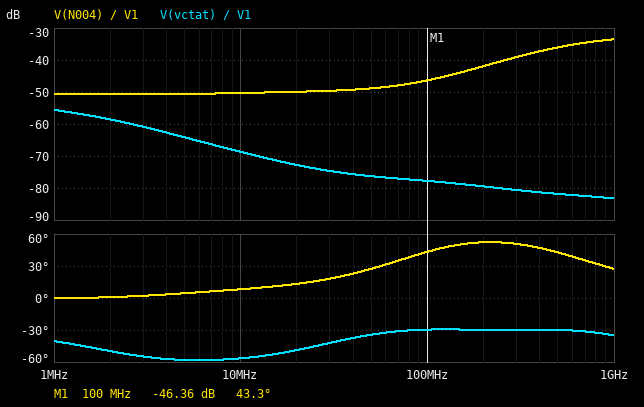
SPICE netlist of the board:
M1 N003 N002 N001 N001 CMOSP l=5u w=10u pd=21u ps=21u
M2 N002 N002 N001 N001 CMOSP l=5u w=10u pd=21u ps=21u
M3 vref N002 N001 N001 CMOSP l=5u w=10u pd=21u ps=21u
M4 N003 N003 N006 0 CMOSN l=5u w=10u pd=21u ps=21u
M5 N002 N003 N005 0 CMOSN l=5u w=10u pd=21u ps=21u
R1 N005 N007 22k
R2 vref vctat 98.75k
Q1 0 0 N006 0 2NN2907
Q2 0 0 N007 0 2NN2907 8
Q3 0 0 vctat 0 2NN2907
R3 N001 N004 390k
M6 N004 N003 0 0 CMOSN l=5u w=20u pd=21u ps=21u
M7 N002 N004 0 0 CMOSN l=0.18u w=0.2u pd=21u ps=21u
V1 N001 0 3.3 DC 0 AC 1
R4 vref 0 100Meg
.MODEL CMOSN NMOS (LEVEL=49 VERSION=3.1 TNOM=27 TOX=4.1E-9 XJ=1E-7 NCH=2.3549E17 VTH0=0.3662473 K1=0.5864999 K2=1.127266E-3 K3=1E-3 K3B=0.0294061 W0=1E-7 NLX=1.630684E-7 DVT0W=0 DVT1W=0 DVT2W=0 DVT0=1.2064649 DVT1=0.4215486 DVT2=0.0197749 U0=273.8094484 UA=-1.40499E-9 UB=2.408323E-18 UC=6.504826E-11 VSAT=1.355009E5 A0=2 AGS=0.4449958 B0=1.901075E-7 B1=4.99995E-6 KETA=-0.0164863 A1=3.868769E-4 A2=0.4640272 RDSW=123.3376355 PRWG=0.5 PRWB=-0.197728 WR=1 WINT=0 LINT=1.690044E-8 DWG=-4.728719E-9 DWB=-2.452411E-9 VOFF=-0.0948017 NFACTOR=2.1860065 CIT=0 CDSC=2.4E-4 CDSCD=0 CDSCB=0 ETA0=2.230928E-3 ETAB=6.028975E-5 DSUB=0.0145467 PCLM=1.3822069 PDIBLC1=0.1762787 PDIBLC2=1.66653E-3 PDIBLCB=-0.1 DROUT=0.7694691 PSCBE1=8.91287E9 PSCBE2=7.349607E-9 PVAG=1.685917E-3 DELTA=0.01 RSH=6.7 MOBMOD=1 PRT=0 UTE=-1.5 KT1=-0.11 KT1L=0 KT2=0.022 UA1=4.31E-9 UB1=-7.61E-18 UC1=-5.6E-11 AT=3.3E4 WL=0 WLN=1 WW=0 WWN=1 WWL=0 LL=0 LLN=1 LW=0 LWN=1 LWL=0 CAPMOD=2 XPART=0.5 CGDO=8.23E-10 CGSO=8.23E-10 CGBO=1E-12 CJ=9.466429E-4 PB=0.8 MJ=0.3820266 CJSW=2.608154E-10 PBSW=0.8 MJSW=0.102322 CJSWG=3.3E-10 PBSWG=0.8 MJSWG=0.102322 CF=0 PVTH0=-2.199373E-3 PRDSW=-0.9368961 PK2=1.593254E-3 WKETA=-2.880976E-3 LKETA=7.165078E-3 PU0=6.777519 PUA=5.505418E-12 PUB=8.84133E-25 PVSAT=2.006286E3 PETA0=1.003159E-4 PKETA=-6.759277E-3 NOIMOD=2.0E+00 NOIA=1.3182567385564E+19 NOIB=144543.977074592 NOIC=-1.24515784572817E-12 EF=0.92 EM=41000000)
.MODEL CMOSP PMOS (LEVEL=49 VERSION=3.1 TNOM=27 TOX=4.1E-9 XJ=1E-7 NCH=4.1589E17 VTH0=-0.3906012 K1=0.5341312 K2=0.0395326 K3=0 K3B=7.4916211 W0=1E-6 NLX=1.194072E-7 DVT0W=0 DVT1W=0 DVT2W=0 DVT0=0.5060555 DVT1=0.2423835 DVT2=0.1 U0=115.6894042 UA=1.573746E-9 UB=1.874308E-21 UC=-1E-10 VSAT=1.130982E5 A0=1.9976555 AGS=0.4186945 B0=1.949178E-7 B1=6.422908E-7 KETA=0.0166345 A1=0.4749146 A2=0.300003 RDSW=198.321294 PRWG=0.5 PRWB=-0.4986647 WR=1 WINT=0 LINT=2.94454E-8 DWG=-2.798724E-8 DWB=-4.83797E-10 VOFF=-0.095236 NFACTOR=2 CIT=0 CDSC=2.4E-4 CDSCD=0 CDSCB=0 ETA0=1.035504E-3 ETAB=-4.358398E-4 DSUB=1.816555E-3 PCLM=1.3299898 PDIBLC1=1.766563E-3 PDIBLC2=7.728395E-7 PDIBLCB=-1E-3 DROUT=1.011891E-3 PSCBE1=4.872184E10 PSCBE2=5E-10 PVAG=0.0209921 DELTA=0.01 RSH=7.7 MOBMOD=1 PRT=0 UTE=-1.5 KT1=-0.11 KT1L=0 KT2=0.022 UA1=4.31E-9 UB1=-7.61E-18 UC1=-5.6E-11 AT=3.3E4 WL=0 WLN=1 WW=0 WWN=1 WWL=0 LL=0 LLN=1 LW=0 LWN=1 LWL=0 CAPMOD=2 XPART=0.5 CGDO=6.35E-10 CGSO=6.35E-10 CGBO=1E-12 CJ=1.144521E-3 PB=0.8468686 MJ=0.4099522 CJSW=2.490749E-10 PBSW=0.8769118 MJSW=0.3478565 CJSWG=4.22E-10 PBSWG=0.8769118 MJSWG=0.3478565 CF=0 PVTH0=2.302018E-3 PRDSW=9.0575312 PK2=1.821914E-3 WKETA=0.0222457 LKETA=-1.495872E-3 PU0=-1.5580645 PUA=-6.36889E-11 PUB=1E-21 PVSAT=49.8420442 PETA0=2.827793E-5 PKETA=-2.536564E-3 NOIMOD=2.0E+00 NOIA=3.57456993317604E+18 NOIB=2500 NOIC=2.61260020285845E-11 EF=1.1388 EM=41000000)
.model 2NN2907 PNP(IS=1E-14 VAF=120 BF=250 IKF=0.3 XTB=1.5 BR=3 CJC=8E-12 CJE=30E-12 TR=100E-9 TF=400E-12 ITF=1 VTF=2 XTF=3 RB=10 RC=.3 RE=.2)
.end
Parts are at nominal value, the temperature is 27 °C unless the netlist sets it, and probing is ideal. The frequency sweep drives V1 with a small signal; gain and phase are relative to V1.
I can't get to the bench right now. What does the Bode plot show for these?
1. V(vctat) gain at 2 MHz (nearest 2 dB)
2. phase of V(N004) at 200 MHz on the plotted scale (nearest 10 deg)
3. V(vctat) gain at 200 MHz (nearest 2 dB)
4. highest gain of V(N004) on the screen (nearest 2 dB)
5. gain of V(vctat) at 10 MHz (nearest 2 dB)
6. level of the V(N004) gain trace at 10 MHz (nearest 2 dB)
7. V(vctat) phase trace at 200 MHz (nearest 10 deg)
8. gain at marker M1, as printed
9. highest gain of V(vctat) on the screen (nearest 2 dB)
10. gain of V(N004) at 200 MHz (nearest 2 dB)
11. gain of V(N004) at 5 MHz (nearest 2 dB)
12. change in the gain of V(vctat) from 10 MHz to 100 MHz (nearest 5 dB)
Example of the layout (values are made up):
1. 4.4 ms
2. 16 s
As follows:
1. -58 dB
2. 50 deg
3. -80 dB
4. -34 dB
5. -68 dB
6. -50 dB
7. -30 deg
8. -46.36 dB
9. -56 dB
10. -42 dB
11. -50 dB
12. -10 dB
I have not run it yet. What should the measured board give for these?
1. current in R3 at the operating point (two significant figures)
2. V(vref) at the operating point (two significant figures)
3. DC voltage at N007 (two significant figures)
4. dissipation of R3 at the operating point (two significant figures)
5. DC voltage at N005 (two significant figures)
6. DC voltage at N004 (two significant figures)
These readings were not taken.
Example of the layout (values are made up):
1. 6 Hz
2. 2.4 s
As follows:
1. 8.4 µA
2. 800 mV
3. 450 mV
4. 28 µW
5. 510 mV
6. 10 mV
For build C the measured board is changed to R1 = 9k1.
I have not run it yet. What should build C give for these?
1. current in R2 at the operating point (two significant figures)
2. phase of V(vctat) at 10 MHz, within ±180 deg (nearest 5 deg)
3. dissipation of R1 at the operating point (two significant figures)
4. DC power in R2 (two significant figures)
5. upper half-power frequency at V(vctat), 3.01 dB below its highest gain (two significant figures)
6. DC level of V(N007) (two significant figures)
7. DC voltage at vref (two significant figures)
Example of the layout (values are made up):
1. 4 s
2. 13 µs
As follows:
1. 6.8 µA
2. -60 deg
3. 390 nW
4. 4.5 µW
5. 840 kHz
6. 470 mV
7. 1.2 V
